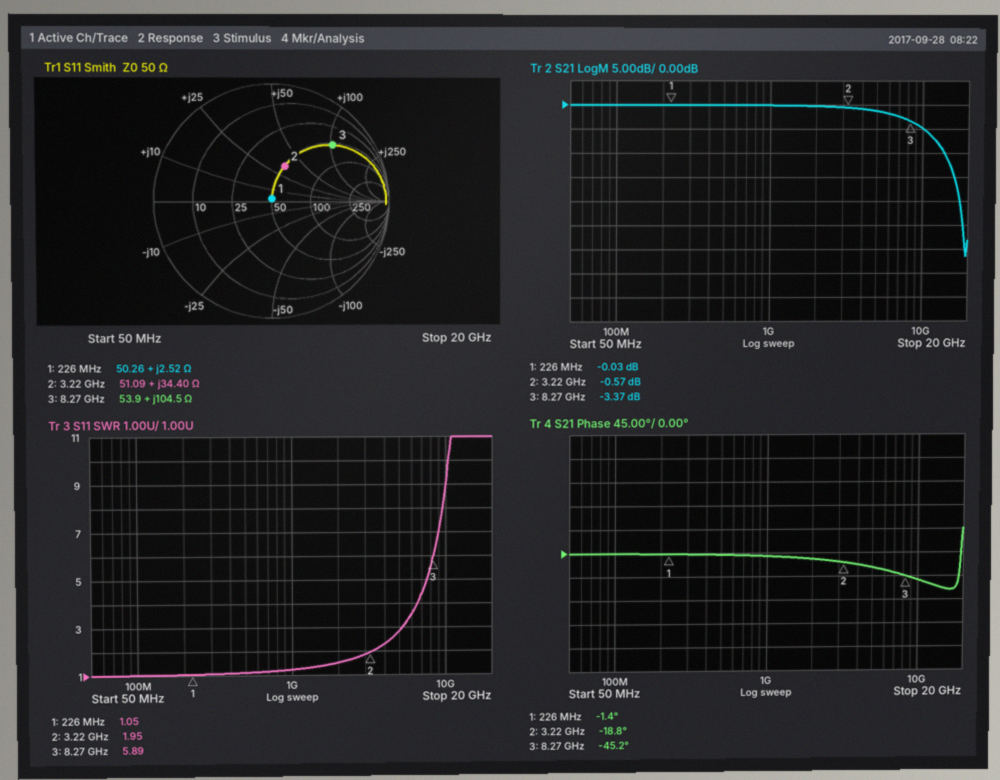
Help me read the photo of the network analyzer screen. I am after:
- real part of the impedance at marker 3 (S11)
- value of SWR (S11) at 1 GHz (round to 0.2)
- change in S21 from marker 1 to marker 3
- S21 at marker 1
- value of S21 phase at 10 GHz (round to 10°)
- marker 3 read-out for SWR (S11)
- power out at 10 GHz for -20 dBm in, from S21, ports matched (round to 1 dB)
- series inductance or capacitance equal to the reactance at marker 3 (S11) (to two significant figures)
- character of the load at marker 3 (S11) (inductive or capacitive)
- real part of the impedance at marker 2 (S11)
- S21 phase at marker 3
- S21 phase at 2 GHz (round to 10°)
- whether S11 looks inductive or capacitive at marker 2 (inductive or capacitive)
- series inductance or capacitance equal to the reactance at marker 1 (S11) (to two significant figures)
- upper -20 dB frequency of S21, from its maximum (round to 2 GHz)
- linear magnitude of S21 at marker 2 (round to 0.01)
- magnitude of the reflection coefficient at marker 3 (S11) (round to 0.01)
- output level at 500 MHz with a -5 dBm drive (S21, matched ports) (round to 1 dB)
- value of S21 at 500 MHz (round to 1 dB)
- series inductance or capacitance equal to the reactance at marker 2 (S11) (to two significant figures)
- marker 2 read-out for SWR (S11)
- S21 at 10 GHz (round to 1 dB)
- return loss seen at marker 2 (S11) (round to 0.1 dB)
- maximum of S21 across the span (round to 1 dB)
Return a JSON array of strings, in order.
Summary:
["53.9 Ω", "1.2", "-3.34 dB", "-0.03 dB", "-50°", "5.89", "-25 dBm", "2.0 nH", "inductive", "51.09 Ω", "-45.2°", "-10°", "inductive", "1.8 nH", "18 GHz", "0.94", "0.71", "-5 dBm", "0 dB", "1.7 nH", "1.95", "-5 dB", "9.8 dB", "0 dB"]
